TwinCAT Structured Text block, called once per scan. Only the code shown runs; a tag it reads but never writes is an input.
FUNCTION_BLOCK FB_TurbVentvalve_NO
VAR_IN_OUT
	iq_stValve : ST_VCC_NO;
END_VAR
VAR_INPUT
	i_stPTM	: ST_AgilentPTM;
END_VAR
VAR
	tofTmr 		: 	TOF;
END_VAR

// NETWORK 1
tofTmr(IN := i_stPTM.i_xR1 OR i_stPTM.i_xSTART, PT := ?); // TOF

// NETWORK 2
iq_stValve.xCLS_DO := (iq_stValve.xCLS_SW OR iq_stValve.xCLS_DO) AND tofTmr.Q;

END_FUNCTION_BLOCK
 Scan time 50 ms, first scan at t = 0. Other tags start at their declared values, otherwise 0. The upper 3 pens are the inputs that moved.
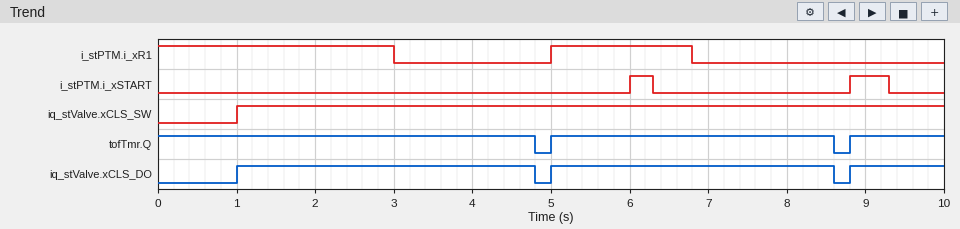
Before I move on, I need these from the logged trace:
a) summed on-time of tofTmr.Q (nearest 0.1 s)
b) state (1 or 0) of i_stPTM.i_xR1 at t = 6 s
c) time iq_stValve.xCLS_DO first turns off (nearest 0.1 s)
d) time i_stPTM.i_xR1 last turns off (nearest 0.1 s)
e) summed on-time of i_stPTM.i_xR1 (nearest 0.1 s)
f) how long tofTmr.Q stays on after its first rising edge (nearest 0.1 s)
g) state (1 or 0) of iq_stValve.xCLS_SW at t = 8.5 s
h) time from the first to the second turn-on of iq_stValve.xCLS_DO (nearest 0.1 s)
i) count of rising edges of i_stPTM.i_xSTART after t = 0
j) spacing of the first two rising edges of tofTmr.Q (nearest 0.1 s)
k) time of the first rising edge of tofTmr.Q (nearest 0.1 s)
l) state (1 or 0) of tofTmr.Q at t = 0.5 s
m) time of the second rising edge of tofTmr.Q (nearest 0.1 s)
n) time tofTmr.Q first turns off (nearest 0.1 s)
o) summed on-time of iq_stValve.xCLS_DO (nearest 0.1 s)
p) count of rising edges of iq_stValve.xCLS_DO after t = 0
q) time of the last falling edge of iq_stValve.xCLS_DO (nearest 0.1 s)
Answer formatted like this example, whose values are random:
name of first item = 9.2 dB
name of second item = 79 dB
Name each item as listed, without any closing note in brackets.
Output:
summed on-time of tofTmr.Q = 9.6 s
state (1 or 0) of i_stPTM.i_xR1 at t = 6 s = 1
time iq_stValve.xCLS_DO first turns off = 4.8 s
time i_stPTM.i_xR1 last turns off = 6.8 s
summed on-time of i_stPTM.i_xR1 = 4.8 s
how long tofTmr.Q stays on after its first rising edge = 3.6 s
state (1 or 0) of iq_stValve.xCLS_SW at t = 8.5 s = 1
time from the first to the second turn-on of iq_stValve.xCLS_DO = 4.0 s
count of rising edges of i_stPTM.i_xSTART after t = 0 = 2
spacing of the first two rising edges of tofTmr.Q = 3.8 s
time of the first rising edge of tofTmr.Q = 5.0 s
state (1 or 0) of tofTmr.Q at t = 0.5 s = 1
time of the second rising edge of tofTmr.Q = 8.8 s
time tofTmr.Q first turns off = 4.8 s
summed on-time of iq_stValve.xCLS_DO = 8.6 s
count of rising edges of iq_stValve.xCLS_DO after t = 0 = 3
time of the last falling edge of iq_stValve.xCLS_DO = 8.6 s
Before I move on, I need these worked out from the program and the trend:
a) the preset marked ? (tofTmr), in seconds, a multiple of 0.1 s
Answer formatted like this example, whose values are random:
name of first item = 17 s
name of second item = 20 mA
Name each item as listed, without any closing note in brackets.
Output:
the preset marked ? (tofTmr), in seconds, a multiple of 0.1 s = 1.8 s
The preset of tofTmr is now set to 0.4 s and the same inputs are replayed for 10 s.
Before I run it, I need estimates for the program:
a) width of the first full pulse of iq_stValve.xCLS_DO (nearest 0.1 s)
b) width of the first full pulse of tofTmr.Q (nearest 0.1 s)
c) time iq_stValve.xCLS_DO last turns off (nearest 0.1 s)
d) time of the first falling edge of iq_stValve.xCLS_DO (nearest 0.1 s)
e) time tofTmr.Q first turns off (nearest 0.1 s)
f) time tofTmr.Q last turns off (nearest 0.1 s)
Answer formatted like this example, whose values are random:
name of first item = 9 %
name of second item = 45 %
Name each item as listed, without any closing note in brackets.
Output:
width of the first full pulse of iq_stValve.xCLS_DO = 2.4 s
width of the first full pulse of tofTmr.Q = 2.2 s
time iq_stValve.xCLS_DO last turns off = 9.7 s
time of the first falling edge of iq_stValve.xCLS_DO = 3.4 s
time tofTmr.Q first turns off = 3.4 s
time tofTmr.Q last turns off = 9.7 s
